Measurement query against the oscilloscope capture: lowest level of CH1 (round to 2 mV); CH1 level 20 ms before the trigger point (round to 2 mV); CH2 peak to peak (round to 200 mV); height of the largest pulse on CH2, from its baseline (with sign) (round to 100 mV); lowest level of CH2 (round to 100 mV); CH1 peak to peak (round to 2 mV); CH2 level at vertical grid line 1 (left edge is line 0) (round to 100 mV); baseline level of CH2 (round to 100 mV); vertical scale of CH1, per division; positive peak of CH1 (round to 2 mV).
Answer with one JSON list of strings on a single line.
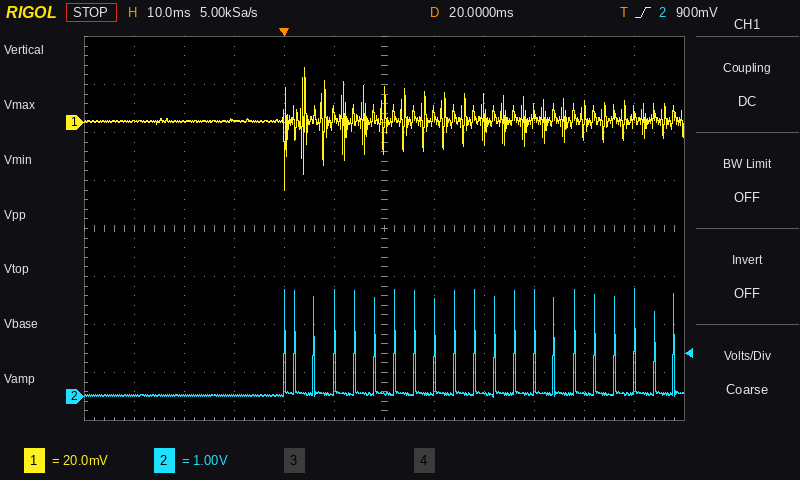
["-28 mV", "0 mV", "2.2 V", "+2.2 V", "0.0 V", "52 mV", "0.0 V", "0.0 V", "20 mV", "24 mV"]
